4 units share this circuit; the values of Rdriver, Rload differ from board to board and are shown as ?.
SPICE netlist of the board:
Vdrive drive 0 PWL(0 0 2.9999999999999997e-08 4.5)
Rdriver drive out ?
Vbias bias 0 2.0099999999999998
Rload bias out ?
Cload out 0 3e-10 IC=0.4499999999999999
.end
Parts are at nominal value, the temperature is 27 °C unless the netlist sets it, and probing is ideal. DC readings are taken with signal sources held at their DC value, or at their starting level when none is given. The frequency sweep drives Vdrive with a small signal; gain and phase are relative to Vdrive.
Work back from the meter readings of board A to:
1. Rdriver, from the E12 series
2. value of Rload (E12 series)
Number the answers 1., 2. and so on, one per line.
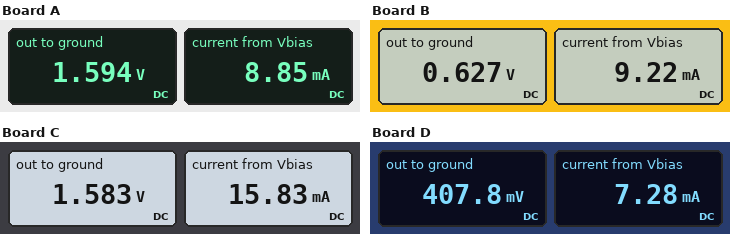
1. 180 Ω
2. 47 Ω
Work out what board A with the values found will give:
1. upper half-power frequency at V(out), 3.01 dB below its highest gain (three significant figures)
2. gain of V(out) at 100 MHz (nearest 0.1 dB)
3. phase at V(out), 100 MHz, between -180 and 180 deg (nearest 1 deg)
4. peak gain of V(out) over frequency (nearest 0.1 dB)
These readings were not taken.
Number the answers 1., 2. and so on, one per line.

1. 14.2 MHz
2. -30.7 dB
3. -82 deg
4. -13.7 dB
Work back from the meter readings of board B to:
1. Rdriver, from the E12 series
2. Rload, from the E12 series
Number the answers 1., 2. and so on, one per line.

1. 68 Ω
2. 150 Ω
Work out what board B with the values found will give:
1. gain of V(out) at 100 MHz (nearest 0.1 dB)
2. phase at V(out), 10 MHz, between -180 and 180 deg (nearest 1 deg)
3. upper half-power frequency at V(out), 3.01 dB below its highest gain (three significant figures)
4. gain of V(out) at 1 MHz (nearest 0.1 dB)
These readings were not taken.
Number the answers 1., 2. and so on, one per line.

1. -22.2 dB
2. -41 deg
3. 11.3 MHz
4. -3.3 dB
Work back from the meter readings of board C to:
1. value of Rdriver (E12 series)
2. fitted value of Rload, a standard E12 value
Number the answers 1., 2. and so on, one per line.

1. 100 Ω
2. 27 Ω
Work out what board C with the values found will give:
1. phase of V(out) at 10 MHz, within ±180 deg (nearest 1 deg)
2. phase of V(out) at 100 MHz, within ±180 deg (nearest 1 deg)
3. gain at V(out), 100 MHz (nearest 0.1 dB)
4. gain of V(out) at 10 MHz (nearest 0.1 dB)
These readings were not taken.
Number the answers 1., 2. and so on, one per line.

1. -22 deg
2. -76 deg
3. -25.8 dB
4. -14.1 dB
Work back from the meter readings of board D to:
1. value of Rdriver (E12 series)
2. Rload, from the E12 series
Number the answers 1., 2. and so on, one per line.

1. 56 Ω
2. 220 Ω
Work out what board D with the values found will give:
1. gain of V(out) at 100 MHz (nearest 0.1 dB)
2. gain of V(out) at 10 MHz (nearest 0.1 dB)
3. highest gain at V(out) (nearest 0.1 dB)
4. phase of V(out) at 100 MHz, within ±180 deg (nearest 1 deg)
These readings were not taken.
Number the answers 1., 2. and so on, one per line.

1. -20.5 dB
2. -4.3 dB
3. -2.0 dB
4. -83 deg
